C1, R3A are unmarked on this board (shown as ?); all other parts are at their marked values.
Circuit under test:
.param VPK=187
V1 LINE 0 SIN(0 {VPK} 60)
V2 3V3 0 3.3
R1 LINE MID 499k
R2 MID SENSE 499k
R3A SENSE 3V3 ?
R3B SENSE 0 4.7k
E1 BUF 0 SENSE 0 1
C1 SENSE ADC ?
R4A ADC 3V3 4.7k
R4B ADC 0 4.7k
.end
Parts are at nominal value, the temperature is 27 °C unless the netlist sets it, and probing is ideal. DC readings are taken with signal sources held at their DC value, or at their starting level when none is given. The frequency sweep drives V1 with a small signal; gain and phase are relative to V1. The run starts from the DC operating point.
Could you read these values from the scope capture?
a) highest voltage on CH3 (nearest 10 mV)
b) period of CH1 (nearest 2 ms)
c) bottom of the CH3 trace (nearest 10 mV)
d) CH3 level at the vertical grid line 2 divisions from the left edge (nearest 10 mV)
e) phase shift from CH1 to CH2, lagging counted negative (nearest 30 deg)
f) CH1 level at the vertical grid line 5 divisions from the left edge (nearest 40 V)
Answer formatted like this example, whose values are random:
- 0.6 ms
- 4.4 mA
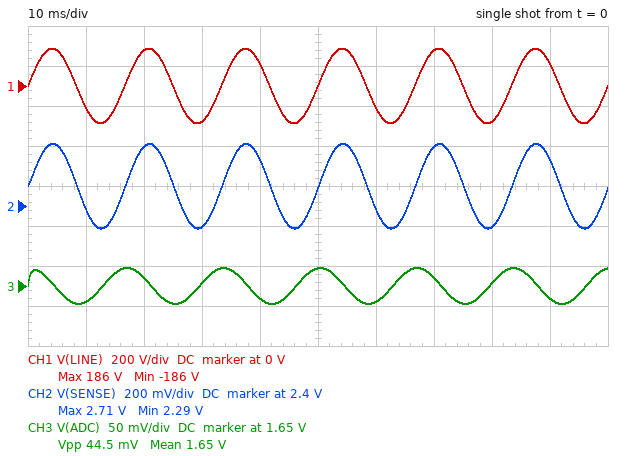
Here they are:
- 1.67 V
- 16 ms
- 1.63 V
- 1.66 V
- 0 deg
- 0 V
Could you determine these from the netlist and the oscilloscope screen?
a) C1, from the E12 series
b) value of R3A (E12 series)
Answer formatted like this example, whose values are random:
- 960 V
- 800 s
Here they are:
- 120 nF
- 1.5 kΩ
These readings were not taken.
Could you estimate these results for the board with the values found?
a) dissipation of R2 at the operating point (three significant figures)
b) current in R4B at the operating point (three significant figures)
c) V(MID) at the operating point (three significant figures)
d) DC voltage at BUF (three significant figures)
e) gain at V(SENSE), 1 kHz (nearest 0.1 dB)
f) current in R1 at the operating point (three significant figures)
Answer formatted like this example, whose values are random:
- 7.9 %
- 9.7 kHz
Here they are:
- 3.13 µW
- 351 µA
- 1.25 V
- 2.50 V
- -61.7 dB
- 2.50 µA
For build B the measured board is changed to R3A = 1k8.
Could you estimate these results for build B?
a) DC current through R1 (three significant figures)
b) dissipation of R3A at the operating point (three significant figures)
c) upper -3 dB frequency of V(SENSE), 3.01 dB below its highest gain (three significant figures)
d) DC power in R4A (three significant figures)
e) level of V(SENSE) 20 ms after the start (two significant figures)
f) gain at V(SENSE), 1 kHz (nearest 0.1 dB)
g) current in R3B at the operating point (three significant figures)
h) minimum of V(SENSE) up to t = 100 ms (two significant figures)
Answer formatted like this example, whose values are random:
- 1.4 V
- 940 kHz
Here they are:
- 2.39 µA
- 467 µW
- 879 Hz
- 579 µW
- 2.6 V
- -60.9 dB
- 507 µA
- 2.1 V
